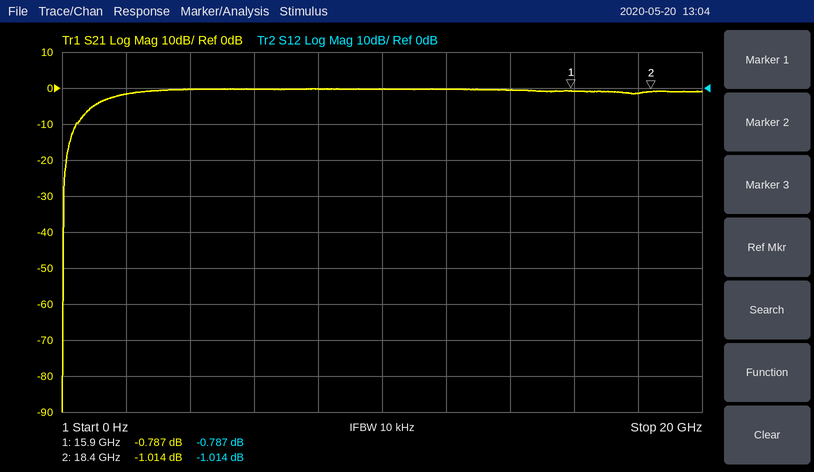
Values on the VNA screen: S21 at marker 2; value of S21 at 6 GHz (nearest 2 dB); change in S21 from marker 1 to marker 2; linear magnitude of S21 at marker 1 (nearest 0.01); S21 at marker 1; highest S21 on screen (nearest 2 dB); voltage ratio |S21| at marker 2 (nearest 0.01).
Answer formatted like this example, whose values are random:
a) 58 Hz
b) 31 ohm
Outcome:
a) -1.014 dB
b) 0 dB
c) -0.227 dB
d) 0.91
e) -0.787 dB
f) 0 dB
g) 0.89
